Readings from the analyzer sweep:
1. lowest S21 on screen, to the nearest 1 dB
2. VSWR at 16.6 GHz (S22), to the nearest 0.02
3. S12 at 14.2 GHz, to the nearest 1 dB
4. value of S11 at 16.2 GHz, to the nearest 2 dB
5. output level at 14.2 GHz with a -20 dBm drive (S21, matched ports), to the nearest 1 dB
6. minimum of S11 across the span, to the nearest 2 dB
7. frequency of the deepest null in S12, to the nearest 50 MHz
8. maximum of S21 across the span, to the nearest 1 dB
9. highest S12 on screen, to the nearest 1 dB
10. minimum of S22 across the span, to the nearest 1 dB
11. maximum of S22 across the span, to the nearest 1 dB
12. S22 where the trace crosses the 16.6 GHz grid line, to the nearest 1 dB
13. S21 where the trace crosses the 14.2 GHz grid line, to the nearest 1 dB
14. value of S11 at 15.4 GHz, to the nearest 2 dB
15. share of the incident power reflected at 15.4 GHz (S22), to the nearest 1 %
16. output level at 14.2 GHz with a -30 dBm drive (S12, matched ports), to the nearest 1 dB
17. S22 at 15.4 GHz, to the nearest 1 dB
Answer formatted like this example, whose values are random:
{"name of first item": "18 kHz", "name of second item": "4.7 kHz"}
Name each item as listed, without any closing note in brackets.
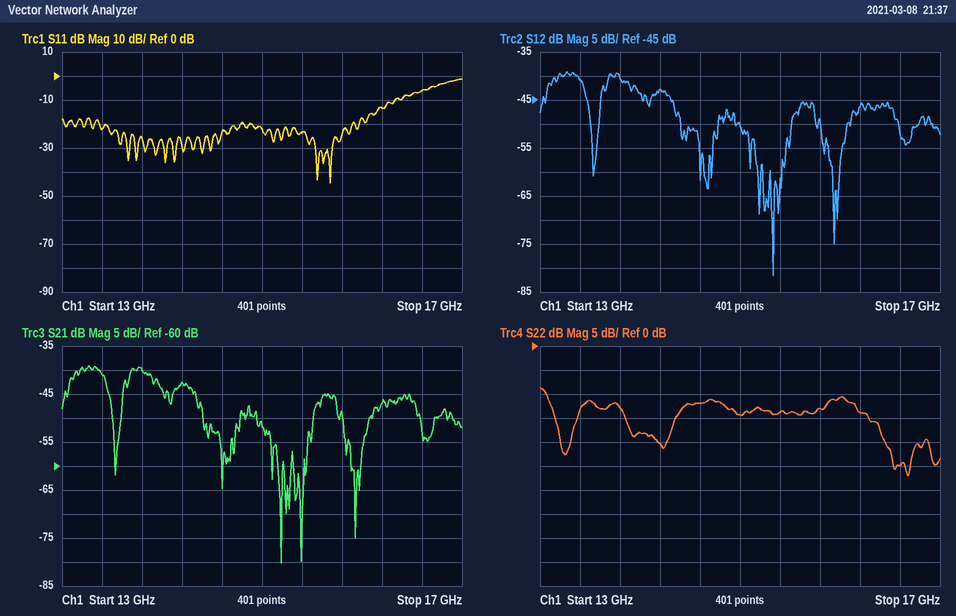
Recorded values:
{"lowest S21 on screen, to the nearest 1 dB": "-80 dB", "VSWR at 16.6 GHz (S22), to the nearest 0.02": "1.12", "S12 at 14.2 GHz, to the nearest 1 dB": "-43 dB", "value of S11 at 16.2 GHz, to the nearest 2 dB": "-14 dB", "output level at 14.2 GHz with a -20 dBm drive (S21, matched ports), to the nearest 1 dB": "-63 dBm", "minimum of S11 across the span, to the nearest 2 dB": "-44 dB", "frequency of the deepest null in S12, to the nearest 50 MHz": "15.35 GHz", "maximum of S21 across the span, to the nearest 1 dB": "-39 dB", "highest S12 on screen, to the nearest 1 dB": "-39 dB", "minimum of S22 across the span, to the nearest 1 dB": "-27 dB", "maximum of S22 across the span, to the nearest 1 dB": "-9 dB", "S22 where the trace crosses the 16.6 GHz grid line, to the nearest 1 dB": "-25 dB", "S21 where the trace crosses the 14.2 GHz grid line, to the nearest 1 dB": "-43 dB", "value of S11 at 15.4 GHz, to the nearest 2 dB": "-24 dB", "share of the incident power reflected at 15.4 GHz (S22), to the nearest 1 %": "4 %", "output level at 14.2 GHz with a -30 dBm drive (S12, matched ports), to the nearest 1 dB": "-73 dBm", "S22 at 15.4 GHz, to the nearest 1 dB": "-14 dB"}
